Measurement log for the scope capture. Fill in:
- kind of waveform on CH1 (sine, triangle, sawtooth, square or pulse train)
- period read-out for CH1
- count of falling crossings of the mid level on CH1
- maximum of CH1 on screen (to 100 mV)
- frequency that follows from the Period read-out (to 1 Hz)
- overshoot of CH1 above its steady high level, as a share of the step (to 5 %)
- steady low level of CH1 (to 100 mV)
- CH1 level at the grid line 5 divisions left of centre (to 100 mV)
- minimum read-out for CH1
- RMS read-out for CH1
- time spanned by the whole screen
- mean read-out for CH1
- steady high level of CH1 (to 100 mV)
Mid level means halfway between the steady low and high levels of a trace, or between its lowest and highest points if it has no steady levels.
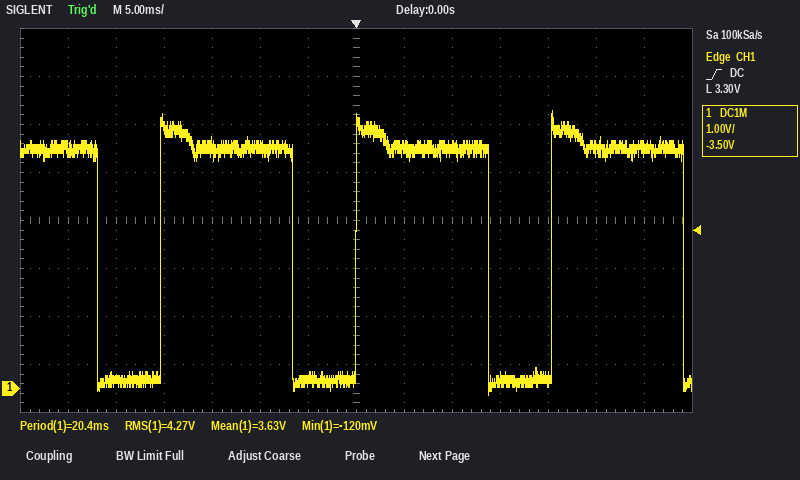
pulse train
20.4 ms
4
5.8 V
49 Hz
15 %
200 mV
200 mV
-120 mV
4.27 V
70 ms
3.63 V
5.0 V
